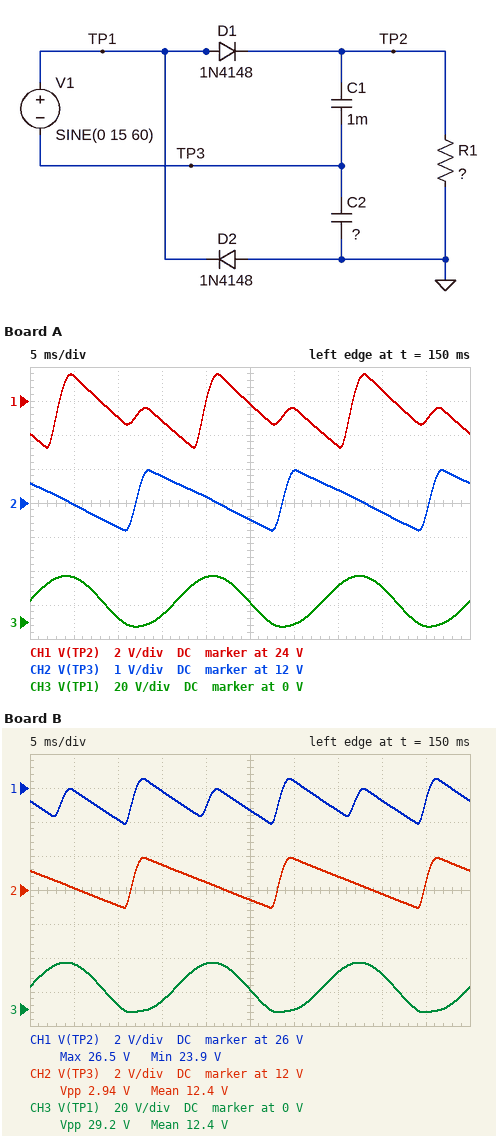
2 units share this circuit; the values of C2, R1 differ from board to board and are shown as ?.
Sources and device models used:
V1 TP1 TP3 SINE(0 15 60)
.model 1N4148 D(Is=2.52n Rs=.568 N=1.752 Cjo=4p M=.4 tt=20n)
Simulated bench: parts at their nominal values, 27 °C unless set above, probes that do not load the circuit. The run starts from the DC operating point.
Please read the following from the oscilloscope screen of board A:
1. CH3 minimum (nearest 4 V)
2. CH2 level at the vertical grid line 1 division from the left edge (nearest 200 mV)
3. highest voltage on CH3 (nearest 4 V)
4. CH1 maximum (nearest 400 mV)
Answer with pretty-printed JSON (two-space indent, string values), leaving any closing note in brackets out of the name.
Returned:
{
  "CH3 minimum": "-4 V",
  "CH2 level at the vertical grid line 1 division from the left edge": "12.0 V",
  "highest voltage on CH3": "28 V",
  "CH1 maximum": "25.6 V"
}
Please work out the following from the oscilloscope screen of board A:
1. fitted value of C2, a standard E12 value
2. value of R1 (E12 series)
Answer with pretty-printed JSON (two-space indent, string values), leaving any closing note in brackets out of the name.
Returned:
{
  "fitted value of C2, a standard E12 value": "2.7 mF",
  "value of R1": "68 Ω"
}
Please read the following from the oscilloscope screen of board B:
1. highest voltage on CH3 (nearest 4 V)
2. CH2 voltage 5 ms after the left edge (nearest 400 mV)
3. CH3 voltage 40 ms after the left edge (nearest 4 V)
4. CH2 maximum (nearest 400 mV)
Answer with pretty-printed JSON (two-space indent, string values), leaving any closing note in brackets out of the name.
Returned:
{
  "highest voltage on CH3": "28 V",
  "CH2 voltage 5 ms after the left edge": "12.0 V",
  "CH3 voltage 40 ms after the left edge": "20 V",
  "CH2 maximum": "14.0 V"
}
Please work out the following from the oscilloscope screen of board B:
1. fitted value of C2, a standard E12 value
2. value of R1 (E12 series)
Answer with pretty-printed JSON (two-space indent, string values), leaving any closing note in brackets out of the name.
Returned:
{
  "fitted value of C2, a standard E12 value": "680 µF",
  "value of R1": "180 Ω"
}
